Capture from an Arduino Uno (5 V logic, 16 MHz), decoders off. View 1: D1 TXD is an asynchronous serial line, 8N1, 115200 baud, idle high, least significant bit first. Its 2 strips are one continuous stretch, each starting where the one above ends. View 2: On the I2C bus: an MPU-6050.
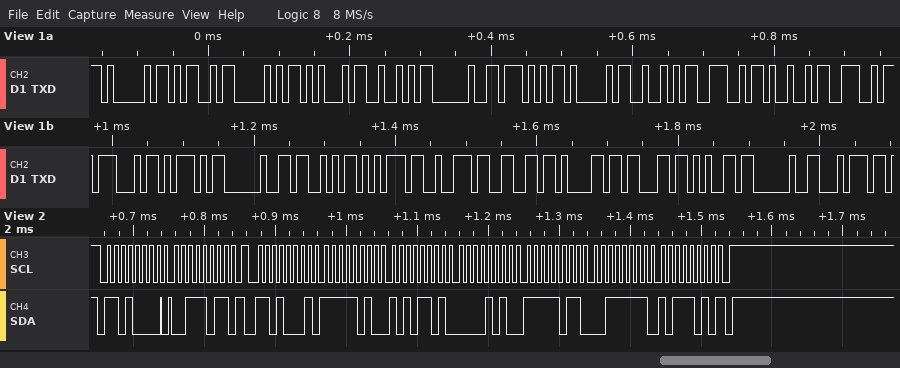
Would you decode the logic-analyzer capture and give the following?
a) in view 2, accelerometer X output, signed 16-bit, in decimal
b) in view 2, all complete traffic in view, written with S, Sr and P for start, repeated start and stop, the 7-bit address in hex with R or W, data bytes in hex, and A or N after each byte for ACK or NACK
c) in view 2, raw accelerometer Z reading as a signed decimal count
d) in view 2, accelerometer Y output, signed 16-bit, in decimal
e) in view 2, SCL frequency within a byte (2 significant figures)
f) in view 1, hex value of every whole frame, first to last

-1363
S 68W A 3B A Sr 68R A FA A AD A 0A A FB A 3F A BA N P
16314
2811
100 kHz
41 4D 50 45 52 20 57 41 52 4E 49 4E 47 5D 20 53 75 72 66 61 63 65 20 74
